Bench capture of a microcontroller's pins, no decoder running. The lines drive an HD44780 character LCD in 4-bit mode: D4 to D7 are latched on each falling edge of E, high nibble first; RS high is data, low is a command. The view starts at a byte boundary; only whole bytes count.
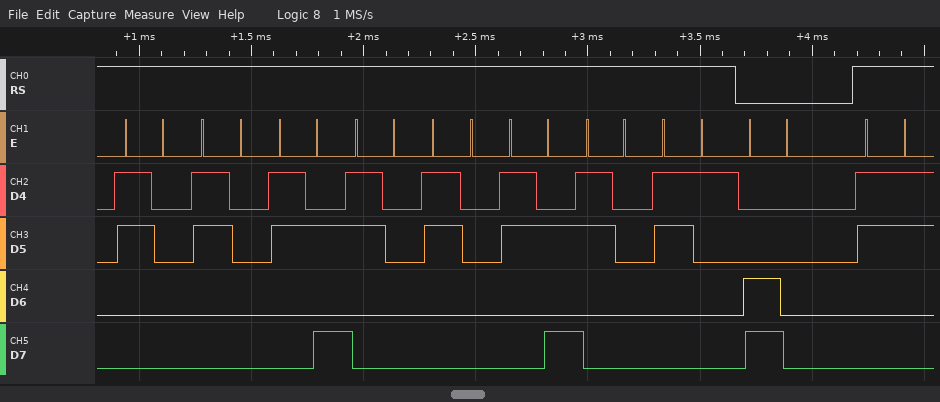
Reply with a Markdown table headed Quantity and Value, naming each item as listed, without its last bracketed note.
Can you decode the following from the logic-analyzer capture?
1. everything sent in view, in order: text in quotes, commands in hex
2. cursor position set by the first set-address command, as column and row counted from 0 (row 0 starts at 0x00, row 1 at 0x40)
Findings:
| Quantity | Value |
|---|---|
| everything sent in view, in order: text in quotes, commands in hex | "00:00:01" 0xC0 "3" |
| cursor position set by the first set-address command, as column and row counted from 0 | column 0, row 1 |
